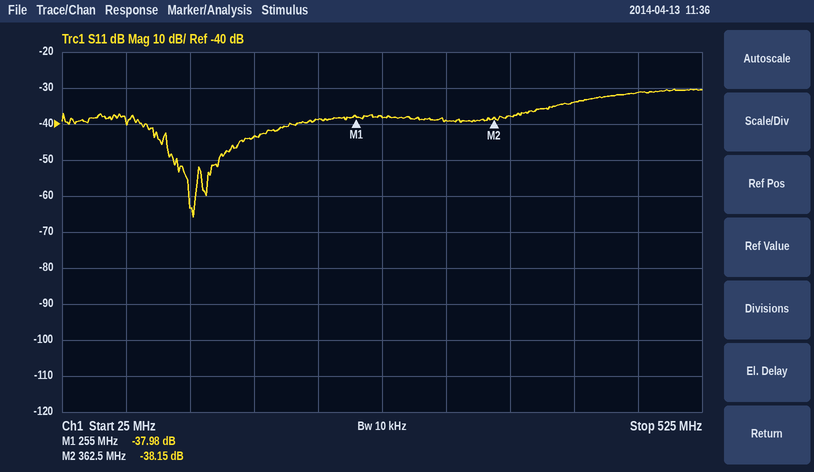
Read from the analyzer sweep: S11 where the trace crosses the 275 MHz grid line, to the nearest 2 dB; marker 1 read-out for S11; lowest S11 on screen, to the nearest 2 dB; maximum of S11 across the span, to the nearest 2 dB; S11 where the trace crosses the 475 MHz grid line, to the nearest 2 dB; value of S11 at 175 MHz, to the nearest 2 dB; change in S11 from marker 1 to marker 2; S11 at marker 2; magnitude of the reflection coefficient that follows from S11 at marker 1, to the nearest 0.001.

-38 dB
-37.98 dB
-66 dB
-30 dB
-32 dB
-44 dB
-0.17 dB
-38.15 dB
0.013
